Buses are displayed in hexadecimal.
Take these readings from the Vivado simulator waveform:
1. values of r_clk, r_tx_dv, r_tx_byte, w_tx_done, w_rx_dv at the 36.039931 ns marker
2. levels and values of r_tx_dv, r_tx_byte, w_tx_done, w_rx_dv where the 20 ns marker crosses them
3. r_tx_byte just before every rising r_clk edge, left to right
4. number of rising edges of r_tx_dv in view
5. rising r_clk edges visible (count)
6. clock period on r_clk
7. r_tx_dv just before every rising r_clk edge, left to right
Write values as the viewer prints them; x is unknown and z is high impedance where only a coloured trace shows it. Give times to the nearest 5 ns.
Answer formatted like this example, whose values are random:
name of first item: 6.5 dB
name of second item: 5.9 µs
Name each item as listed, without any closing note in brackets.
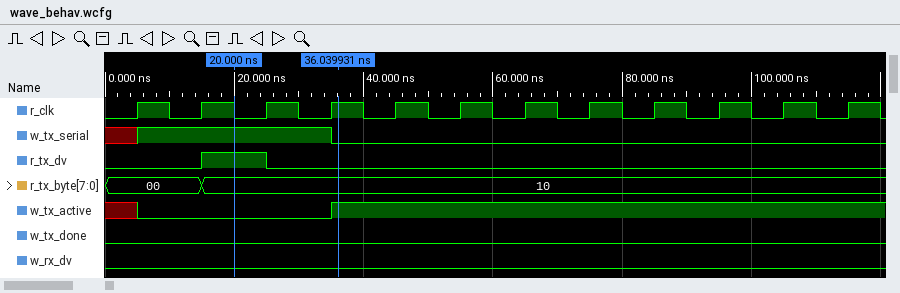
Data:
values of r_clk, r_tx_dv, r_tx_byte, w_tx_done, w_rx_dv at the 36.039931 ns marker: r_clk=1, r_tx_dv=0, r_tx_byte=10, w_tx_done=0, w_rx_dv=0
levels and values of r_tx_dv, r_tx_byte, w_tx_done, w_rx_dv where the 20 ns marker crosses them: r_tx_dv=1, r_tx_byte=10, w_tx_done=0, w_rx_dv=0
r_tx_byte just before every rising r_clk edge, left to right: 00, 00, 10, 10, 10, 10, 10, 10, 10, 10, 10, 10
number of rising edges of r_tx_dv in view: 1
rising r_clk edges visible: 12
clock period on r_clk: 10 ns
r_tx_dv just before every rising r_clk edge, left to right: 0 0 1 0 0 0 0 0 0 0 0 0
